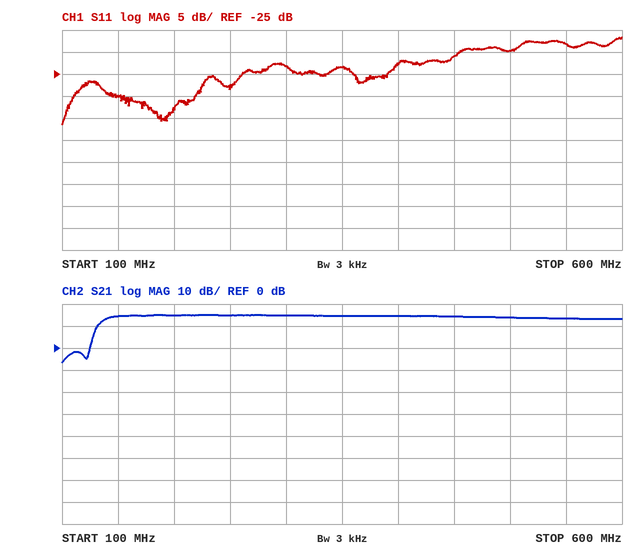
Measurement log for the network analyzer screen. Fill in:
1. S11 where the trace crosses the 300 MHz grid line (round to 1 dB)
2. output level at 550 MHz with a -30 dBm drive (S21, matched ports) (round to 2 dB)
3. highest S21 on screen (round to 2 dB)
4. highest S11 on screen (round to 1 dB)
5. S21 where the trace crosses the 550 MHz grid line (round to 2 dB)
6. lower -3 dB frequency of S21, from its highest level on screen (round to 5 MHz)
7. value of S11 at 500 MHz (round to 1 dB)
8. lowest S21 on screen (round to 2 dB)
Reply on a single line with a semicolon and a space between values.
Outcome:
-23 dB; -16 dBm; 16 dB; -17 dB; 14 dB; 135 MHz; -20 dB; -6 dB
